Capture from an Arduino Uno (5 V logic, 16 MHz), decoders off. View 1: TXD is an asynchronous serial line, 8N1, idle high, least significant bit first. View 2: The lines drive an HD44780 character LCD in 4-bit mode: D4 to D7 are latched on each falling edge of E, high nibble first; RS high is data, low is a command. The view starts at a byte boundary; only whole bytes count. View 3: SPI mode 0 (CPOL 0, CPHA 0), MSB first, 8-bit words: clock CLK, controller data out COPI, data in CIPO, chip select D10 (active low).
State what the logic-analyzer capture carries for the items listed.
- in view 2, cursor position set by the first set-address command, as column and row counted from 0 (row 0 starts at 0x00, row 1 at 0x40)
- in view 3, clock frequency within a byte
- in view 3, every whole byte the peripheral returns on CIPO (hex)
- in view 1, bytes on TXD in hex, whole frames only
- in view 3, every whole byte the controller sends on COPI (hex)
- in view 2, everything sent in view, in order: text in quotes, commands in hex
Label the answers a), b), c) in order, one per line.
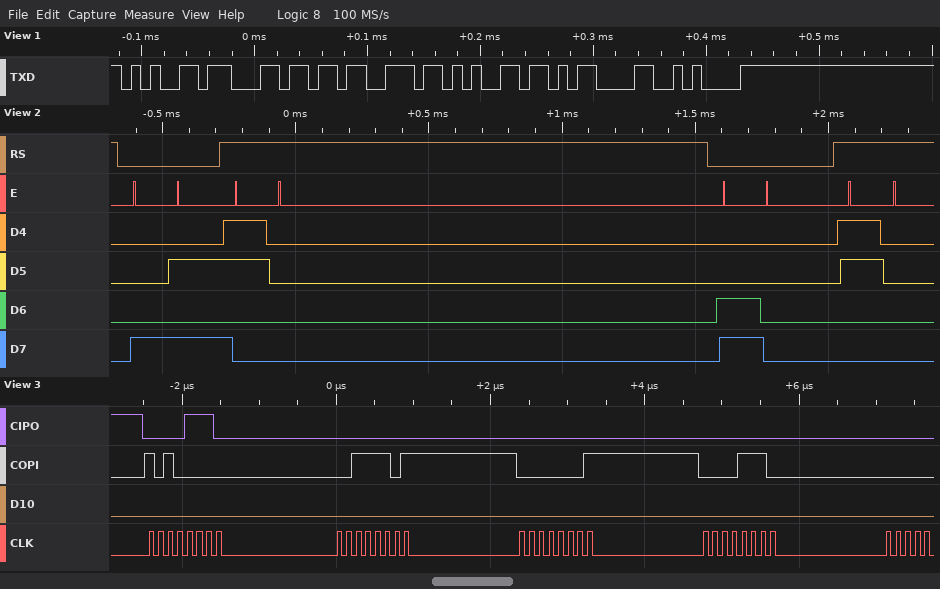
a) column 10, row 0
b) 8 MHz
c) 0E 00 00 00
d) 0x65 0x6C 0x73 0x65 0x0D 0x0A
e) A0 3D 01 0E
f) 0x8A "0" 0xC0 "0"
